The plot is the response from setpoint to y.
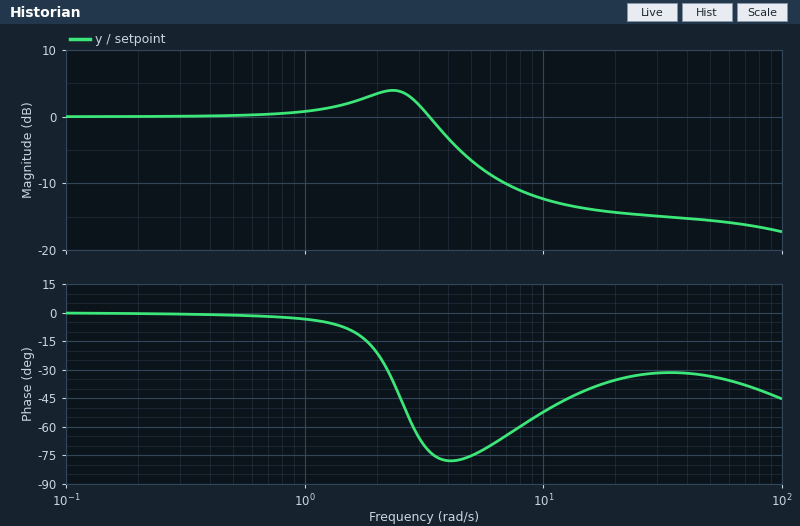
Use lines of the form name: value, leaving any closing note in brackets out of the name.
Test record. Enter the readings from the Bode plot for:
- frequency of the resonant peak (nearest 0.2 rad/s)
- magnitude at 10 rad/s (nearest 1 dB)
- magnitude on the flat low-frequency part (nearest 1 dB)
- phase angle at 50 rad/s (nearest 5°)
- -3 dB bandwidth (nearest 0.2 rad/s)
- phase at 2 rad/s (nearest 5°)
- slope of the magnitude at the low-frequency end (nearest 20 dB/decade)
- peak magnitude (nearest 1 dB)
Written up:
frequency of the resonant peak: 2.4 rad/s
magnitude at 10 rad/s: -12 dB
magnitude on the flat low-frequency part: 0 dB
phase angle at 50 rad/s: -35°
-3 dB bandwidth: 4.0 rad/s
phase at 2 rad/s: -20°
slope of the magnitude at the low-frequency end: 0 dB/decade
peak magnitude: 4 dB
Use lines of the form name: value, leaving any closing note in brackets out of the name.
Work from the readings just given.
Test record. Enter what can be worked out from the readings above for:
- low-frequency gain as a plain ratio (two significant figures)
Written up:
low-frequency gain as a plain ratio: 1.0
